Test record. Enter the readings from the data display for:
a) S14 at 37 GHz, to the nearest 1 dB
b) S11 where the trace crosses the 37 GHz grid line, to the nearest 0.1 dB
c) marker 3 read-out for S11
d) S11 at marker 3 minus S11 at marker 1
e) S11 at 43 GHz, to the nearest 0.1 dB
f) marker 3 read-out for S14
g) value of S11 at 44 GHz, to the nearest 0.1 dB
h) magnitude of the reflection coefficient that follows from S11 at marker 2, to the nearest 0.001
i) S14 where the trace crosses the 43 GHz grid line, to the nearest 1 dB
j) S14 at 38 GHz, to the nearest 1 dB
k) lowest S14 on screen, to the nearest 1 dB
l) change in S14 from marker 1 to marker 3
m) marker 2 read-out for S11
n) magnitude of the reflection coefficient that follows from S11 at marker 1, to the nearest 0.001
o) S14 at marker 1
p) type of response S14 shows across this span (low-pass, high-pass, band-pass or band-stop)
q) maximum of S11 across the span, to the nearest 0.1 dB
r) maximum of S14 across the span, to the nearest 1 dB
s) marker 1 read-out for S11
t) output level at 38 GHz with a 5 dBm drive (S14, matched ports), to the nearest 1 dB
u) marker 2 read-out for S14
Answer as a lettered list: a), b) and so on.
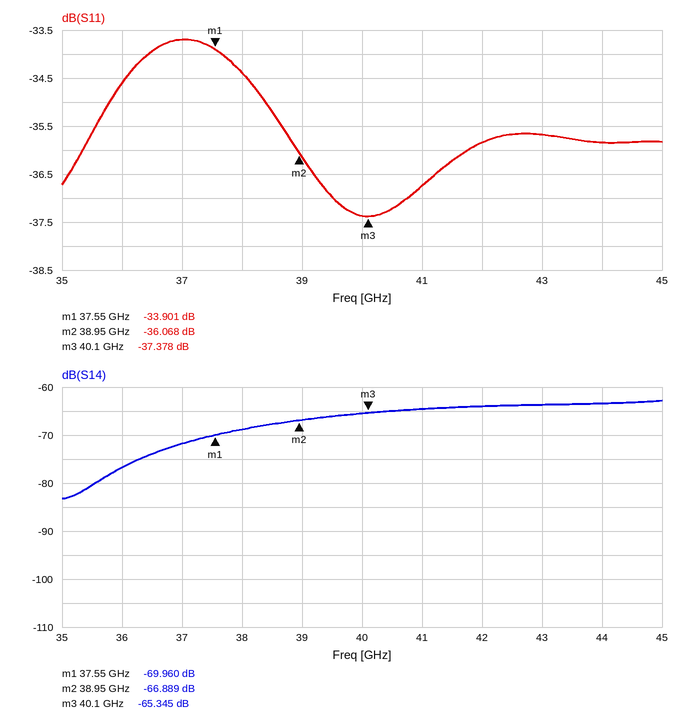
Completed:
a) -72 dB
b) -33.7 dB
c) -37.378 dB
d) -3.477 dB
e) -35.7 dB
f) -65.345 dB
g) -35.8 dB
h) 0.016
i) -64 dB
j) -69 dB
k) -83 dB
l) 4.615 dB
m) -36.068 dB
n) 0.020
o) -69.960 dB
p) high-pass
q) -33.7 dB
r) -63 dB
s) -33.901 dB
t) -64 dBm
u) -66.889 dB
